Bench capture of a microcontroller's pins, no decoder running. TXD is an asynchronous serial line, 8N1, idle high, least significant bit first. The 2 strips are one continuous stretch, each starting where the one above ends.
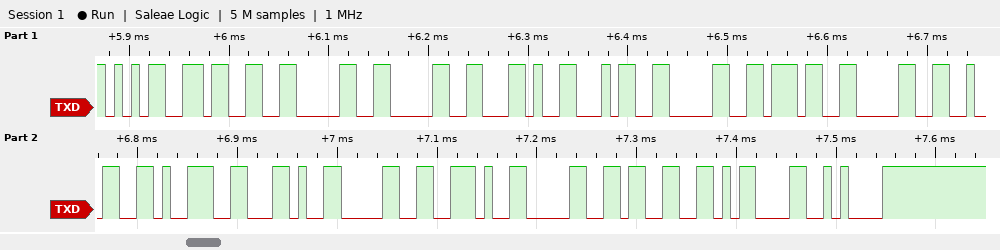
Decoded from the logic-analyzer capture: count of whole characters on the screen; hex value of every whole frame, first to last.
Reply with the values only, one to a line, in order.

18
35 33 30 30 2C 34 30 37 30 32 39 2C 30 2E 30 33 0D 0A
